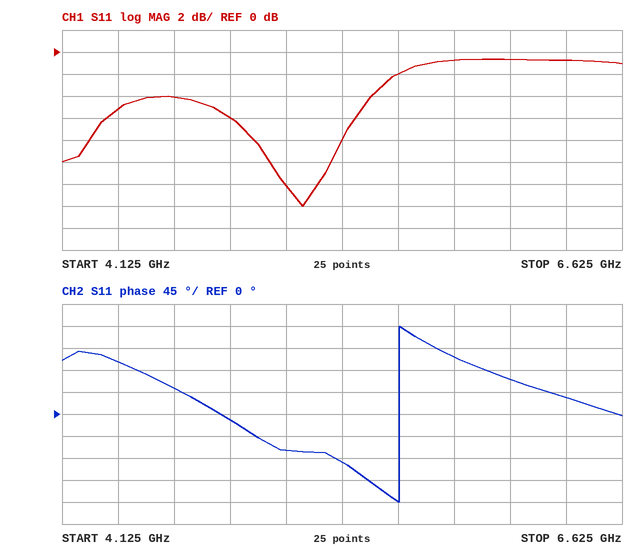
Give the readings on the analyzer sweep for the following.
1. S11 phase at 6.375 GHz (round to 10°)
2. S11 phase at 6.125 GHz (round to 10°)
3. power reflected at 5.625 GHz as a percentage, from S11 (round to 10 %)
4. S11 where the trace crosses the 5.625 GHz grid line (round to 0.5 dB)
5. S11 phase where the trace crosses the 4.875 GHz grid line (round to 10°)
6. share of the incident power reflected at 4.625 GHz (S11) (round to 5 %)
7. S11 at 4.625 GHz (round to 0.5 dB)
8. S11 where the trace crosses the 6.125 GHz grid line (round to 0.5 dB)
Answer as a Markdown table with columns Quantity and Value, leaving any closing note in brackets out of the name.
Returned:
| Quantity | Value |
|---|---|
| S11 phase at 6.375 GHz | 30° |
| S11 phase at 6.125 GHz | 70° |
| power reflected at 5.625 GHz as a percentage, from S11 | 60 % |
| S11 where the trace crosses the 5.625 GHz grid line | -2.0 dB |
| S11 phase where the trace crosses the 4.875 GHz grid line | -10° |
| share of the incident power reflected at 4.625 GHz (S11) | 40 % |
| S11 at 4.625 GHz | -4.0 dB |
| S11 where the trace crosses the 6.125 GHz grid line | -0.5 dB |
